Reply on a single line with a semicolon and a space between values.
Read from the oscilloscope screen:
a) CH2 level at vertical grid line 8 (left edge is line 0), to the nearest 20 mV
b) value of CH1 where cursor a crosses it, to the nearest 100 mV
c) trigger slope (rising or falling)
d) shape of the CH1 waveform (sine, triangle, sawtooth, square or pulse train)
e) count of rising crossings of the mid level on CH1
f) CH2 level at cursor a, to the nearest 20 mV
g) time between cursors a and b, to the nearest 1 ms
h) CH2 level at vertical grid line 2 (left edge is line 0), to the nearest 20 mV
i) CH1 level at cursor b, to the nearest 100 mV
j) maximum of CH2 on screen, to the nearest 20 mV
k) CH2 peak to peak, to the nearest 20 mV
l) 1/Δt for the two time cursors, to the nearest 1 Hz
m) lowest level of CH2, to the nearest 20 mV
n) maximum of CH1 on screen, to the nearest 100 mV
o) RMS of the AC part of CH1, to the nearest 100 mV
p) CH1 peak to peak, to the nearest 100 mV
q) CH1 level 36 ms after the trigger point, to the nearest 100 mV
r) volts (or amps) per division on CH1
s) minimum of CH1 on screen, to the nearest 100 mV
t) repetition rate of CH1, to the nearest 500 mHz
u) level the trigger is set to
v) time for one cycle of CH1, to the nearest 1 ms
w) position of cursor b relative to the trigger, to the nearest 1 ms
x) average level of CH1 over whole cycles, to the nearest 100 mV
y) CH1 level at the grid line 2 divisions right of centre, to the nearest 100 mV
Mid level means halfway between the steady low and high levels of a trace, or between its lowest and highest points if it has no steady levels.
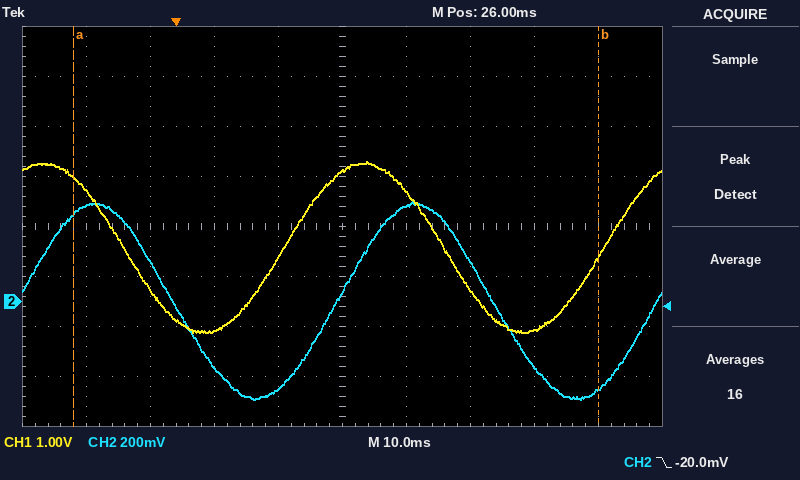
-260 mV; 2.5 V; falling; sine; 2; 340 mV; 82 ms; 160 mV; 900 mV; 400 mV; 800 mV; 12 Hz; -400 mV; 2.8 V; 1.2 V; 3.4 V; 2.2 V; 1 V; -600 mV; 20.0 Hz; -20.0 mV; 50 ms; +66 ms; 1.1 V; 200 mV
